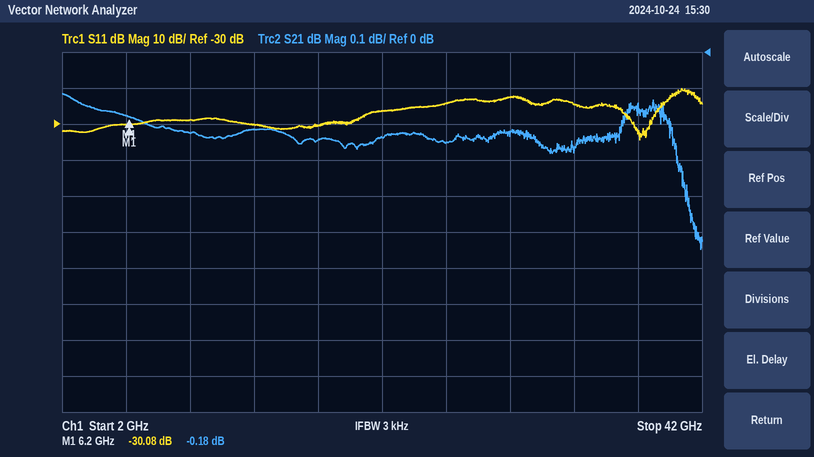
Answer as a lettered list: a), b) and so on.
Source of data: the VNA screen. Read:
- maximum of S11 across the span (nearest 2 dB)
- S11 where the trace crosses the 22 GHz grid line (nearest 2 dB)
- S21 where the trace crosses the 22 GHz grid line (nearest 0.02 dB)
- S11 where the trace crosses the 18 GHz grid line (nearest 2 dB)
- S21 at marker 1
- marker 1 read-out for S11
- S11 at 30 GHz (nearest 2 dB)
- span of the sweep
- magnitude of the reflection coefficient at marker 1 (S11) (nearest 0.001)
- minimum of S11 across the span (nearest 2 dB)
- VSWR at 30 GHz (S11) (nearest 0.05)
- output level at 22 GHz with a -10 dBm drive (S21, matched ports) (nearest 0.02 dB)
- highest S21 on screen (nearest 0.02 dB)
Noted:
a) -20 dB
b) -26 dB
c) -0.24 dB
d) -30 dB
e) -0.18 dB
f) -30.08 dB
g) -22 dB
h) 40 GHz
i) 0.031
j) -34 dB
k) 1.15
l) -10.24 dBm
m) -0.12 dB
